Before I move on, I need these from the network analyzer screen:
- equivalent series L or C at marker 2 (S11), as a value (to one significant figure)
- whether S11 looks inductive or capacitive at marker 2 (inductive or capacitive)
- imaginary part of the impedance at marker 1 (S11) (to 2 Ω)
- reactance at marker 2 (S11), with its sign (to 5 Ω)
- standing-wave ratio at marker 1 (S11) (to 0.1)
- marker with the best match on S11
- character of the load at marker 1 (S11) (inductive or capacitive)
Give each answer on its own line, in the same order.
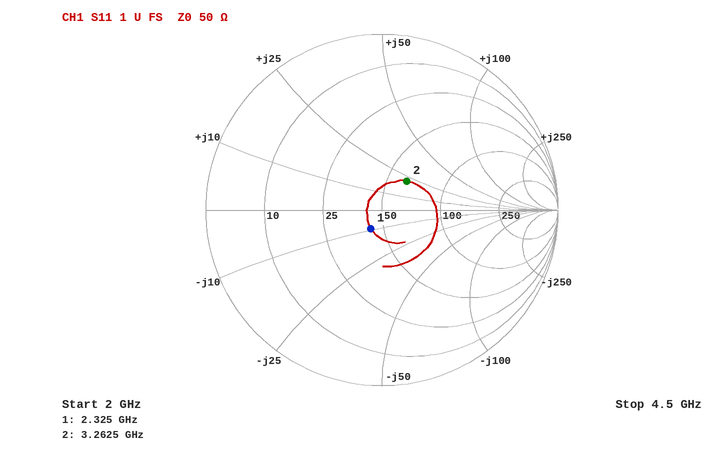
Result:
1 nH
inductive
-10 Ω
+20 Ω
1.3
marker 1
capacitive
